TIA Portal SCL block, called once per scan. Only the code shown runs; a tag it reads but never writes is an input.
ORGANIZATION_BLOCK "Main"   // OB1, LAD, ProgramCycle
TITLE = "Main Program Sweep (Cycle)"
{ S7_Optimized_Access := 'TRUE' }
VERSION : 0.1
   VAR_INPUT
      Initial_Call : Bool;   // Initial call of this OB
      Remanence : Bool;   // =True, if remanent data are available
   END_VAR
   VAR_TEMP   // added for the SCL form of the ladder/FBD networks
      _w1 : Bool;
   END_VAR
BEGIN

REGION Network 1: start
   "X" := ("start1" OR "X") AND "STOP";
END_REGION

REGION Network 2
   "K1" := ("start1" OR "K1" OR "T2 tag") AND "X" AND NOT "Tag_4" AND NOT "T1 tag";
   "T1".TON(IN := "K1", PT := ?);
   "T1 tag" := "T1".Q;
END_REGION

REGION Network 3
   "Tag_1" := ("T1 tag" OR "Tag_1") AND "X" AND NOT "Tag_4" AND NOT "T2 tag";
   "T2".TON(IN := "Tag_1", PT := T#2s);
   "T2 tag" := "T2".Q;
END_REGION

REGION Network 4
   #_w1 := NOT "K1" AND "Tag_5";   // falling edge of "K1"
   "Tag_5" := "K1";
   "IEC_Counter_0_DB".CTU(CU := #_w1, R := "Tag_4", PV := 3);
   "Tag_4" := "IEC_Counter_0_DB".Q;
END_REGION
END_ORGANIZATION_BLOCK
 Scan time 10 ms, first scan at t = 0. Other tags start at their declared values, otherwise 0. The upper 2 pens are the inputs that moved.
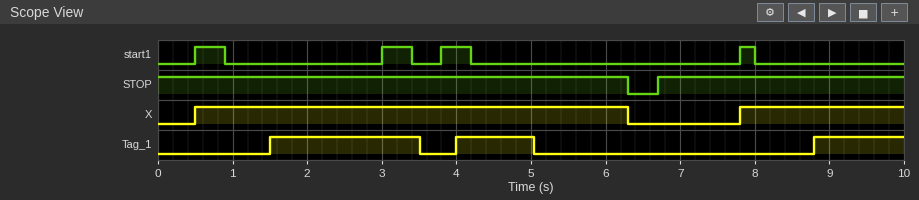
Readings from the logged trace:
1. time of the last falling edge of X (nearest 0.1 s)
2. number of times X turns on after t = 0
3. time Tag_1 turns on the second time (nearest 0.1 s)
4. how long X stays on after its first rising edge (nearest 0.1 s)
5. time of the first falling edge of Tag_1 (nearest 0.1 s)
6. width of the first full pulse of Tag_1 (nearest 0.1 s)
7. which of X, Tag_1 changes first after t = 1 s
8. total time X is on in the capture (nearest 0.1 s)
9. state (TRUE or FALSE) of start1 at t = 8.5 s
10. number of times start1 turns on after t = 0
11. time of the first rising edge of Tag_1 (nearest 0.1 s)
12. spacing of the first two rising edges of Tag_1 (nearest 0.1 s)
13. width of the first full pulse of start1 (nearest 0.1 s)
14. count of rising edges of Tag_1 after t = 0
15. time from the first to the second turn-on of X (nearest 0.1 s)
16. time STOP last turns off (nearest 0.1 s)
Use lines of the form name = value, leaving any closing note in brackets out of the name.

time of the last falling edge of X = 6.3 s
number of times X turns on after t = 0 = 2
time Tag_1 turns on the second time = 4.0 s
how long X stays on after its first rising edge = 5.8 s
time of the first falling edge of Tag_1 = 3.5 s
width of the first full pulse of Tag_1 = 2.0 s
which of X, Tag_1 changes first after t = 1 s = Tag_1
total time X is on in the capture = 8.0 s
state (TRUE or FALSE) of start1 at t = 8.5 s = FALSE
number of times start1 turns on after t = 0 = 4
time of the first rising edge of Tag_1 = 1.5 s
spacing of the first two rising edges of Tag_1 = 2.5 s
width of the first full pulse of start1 = 0.4 s
count of rising edges of Tag_1 after t = 0 = 3
time from the first to the second turn-on of X = 7.3 s
time STOP last turns off = 6.3 s
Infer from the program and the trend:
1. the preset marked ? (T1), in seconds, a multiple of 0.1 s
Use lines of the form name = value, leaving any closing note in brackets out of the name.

the preset marked ? (T1), in seconds, a multiple of 0.1 s = 1.0 s
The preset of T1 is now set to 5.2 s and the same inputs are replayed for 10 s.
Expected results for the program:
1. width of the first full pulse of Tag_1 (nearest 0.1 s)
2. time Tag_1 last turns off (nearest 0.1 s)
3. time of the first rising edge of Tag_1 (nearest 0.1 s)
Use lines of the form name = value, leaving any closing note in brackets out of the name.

width of the first full pulse of Tag_1 = 0.6 s
time Tag_1 last turns off = 6.3 s
time of the first rising edge of Tag_1 = 5.7 s
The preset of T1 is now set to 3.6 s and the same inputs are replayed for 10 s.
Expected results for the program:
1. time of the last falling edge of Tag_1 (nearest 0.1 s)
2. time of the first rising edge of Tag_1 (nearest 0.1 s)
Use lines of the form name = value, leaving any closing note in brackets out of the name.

time of the last falling edge of Tag_1 = 6.1 s
time of the first rising edge of Tag_1 = 4.1 s
